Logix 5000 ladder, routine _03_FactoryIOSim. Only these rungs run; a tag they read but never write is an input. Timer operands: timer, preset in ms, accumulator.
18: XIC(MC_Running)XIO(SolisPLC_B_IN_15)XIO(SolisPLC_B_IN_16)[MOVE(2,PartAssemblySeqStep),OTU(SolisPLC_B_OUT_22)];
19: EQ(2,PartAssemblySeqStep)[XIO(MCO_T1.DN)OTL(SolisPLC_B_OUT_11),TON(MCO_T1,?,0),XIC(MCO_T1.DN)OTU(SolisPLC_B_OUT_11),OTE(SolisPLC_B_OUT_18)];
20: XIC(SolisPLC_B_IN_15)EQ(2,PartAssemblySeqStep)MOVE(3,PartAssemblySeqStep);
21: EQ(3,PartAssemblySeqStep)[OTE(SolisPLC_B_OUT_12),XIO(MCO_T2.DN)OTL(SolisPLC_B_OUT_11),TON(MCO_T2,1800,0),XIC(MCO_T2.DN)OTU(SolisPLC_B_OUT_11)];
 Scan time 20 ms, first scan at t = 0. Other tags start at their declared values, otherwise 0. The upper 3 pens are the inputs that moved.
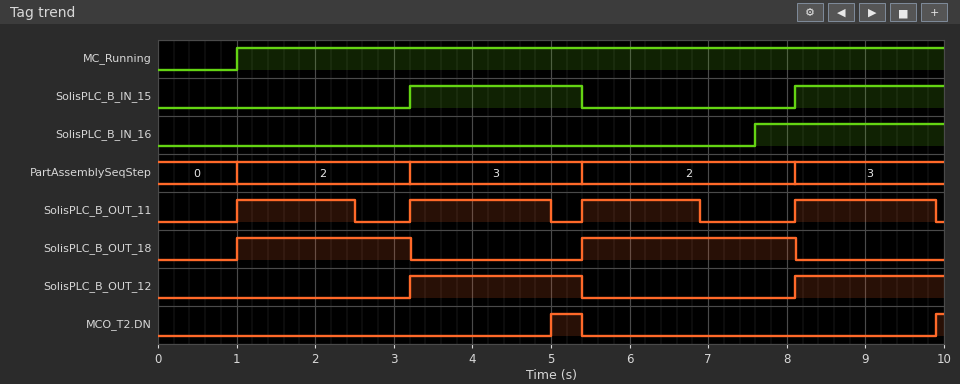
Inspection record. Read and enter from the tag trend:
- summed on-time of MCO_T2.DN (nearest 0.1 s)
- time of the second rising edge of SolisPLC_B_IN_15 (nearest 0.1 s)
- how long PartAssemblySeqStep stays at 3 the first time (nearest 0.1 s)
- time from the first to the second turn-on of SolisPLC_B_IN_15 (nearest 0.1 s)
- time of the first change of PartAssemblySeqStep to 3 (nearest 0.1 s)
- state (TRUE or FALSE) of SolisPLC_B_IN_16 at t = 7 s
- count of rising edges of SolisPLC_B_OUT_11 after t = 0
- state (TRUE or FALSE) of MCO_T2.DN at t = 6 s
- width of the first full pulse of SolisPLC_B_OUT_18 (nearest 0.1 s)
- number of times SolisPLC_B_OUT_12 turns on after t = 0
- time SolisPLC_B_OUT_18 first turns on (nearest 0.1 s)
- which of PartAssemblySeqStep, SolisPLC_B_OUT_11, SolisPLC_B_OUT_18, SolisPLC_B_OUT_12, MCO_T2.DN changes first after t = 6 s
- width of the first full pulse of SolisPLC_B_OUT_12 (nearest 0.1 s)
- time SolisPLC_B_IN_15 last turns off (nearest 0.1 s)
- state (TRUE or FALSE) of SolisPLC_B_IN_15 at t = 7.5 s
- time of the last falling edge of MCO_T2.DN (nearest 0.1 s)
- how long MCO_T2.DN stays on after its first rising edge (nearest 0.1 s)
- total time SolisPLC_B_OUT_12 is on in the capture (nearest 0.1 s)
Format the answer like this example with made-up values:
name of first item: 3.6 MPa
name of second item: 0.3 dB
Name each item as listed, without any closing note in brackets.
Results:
summed on-time of MCO_T2.DN: 0.5 s
time of the second rising edge of SolisPLC_B_IN_15: 8.1 s
how long PartAssemblySeqStep stays at 3 the first time: 2.2 s
time from the first to the second turn-on of SolisPLC_B_IN_15: 4.9 s
time of the first change of PartAssemblySeqStep to 3: 3.2 s
state (TRUE or FALSE) of SolisPLC_B_IN_16 at t = 7 s: FALSE
count of rising edges of SolisPLC_B_OUT_11 after t = 0: 4
state (TRUE or FALSE) of MCO_T2.DN at t = 6 s: FALSE
width of the first full pulse of SolisPLC_B_OUT_18: 2.2 s
number of times SolisPLC_B_OUT_12 turns on after t = 0: 2
time SolisPLC_B_OUT_18 first turns on: 1.0 s
which of PartAssemblySeqStep, SolisPLC_B_OUT_11, SolisPLC_B_OUT_18, SolisPLC_B_OUT_12, MCO_T2.DN changes first after t = 6 s: SolisPLC_B_OUT_11
width of the first full pulse of SolisPLC_B_OUT_12: 2.2 s
time SolisPLC_B_IN_15 last turns off: 5.4 s
state (TRUE or FALSE) of SolisPLC_B_IN_15 at t = 7.5 s: FALSE
time of the last falling edge of MCO_T2.DN: 5.4 s
how long MCO_T2.DN stays on after its first rising edge: 0.4 s
total time SolisPLC_B_OUT_12 is on in the capture: 4.1 s
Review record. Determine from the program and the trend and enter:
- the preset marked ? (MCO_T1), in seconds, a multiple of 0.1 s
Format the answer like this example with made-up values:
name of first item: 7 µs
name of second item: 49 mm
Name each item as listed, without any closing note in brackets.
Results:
the preset marked ? (MCO_T1), in seconds, a multiple of 0.1 s: 1.5 s
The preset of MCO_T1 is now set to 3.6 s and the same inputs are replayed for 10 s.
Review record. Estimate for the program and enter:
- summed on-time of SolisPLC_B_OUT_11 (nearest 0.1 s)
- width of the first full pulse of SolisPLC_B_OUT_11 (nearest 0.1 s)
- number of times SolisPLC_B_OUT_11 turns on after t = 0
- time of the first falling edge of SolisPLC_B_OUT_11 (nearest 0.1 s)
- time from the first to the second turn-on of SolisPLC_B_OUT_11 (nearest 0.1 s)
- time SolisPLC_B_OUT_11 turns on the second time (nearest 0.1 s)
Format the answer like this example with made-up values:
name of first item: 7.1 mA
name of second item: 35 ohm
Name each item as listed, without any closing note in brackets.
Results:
summed on-time of SolisPLC_B_OUT_11: 8.5 s
width of the first full pulse of SolisPLC_B_OUT_11: 4.0 s
number of times SolisPLC_B_OUT_11 turns on after t = 0: 2
time of the first falling edge of SolisPLC_B_OUT_11: 5.0 s
time from the first to the second turn-on of SolisPLC_B_OUT_11: 4.4 s
time SolisPLC_B_OUT_11 turns on the second time: 5.4 s
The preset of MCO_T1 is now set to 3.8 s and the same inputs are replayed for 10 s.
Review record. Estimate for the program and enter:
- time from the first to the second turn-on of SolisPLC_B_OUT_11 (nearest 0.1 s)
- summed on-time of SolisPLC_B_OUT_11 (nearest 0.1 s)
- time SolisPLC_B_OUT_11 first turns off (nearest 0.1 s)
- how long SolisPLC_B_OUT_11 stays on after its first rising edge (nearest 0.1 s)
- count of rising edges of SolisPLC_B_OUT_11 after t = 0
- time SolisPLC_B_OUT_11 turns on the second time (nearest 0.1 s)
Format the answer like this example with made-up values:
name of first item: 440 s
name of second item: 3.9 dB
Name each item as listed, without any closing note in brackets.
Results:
time from the first to the second turn-on of SolisPLC_B_OUT_11: 4.4 s
summed on-time of SolisPLC_B_OUT_11: 8.5 s
time SolisPLC_B_OUT_11 first turns off: 5.0 s
how long SolisPLC_B_OUT_11 stays on after its first rising edge: 4.0 s
count of rising edges of SolisPLC_B_OUT_11 after t = 0: 2
time SolisPLC_B_OUT_11 turns on the second time: 5.4 s
